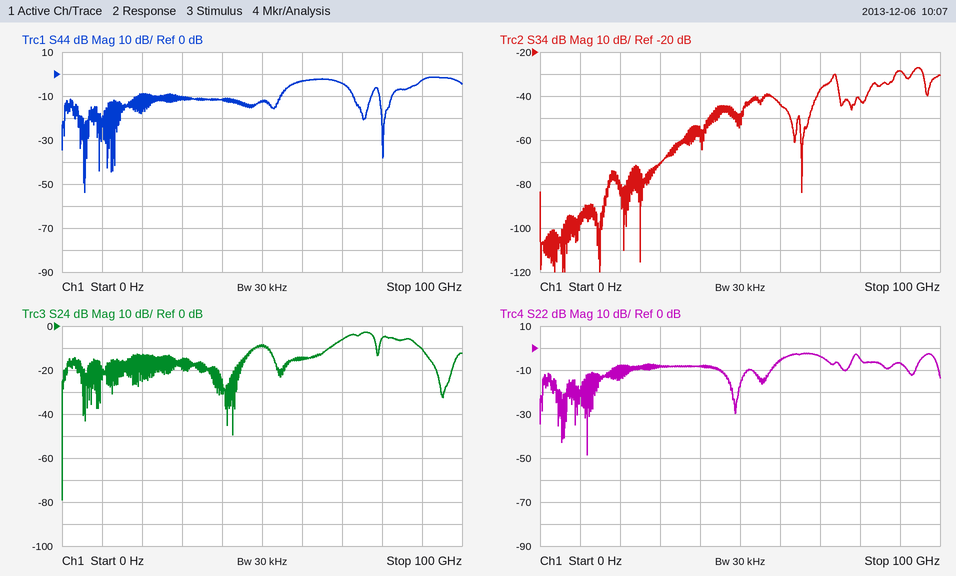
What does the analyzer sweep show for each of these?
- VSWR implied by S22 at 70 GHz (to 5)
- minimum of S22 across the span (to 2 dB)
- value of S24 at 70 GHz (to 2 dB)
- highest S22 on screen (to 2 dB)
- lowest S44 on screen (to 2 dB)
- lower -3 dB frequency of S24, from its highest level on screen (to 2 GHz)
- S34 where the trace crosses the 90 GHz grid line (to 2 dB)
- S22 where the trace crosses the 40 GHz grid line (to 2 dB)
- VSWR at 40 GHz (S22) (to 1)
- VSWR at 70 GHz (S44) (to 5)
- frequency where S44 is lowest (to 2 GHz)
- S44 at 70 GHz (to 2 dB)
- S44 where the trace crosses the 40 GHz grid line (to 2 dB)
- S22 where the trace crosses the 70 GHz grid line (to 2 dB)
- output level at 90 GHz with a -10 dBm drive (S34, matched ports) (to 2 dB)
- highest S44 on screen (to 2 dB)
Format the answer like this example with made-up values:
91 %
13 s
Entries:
5
-48 dB
-6 dB
-2 dB
-54 dB
70 GHz
-28 dB
-8 dB
2
5
6 GHz
-4 dB
-12 dB
-4 dB
-38 dBm
-2 dB
